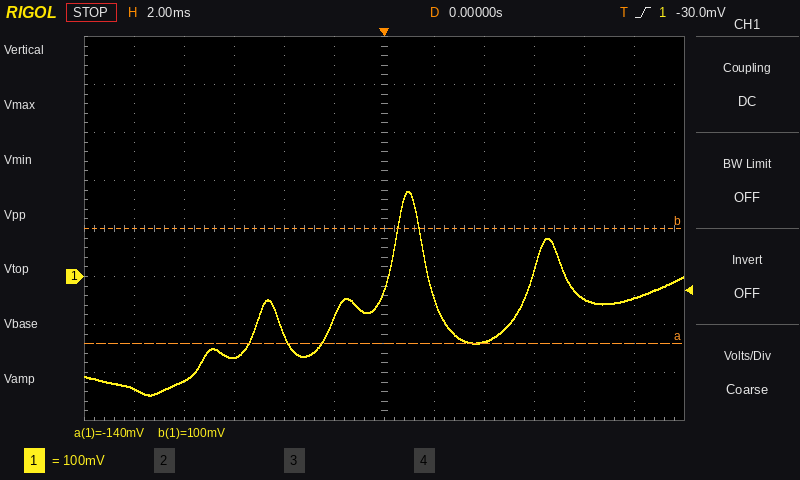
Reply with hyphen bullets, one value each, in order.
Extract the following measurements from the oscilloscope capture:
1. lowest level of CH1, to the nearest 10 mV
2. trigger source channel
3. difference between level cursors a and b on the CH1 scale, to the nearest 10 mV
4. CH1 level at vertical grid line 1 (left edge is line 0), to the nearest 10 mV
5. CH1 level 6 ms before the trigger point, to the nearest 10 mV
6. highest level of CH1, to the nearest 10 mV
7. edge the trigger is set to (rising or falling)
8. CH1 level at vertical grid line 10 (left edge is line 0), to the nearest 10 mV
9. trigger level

- -250 mV
- CH1
- 240 mV
- -230 mV
- -170 mV
- 180 mV
- rising
- -50 mV
- -30.0 mV
